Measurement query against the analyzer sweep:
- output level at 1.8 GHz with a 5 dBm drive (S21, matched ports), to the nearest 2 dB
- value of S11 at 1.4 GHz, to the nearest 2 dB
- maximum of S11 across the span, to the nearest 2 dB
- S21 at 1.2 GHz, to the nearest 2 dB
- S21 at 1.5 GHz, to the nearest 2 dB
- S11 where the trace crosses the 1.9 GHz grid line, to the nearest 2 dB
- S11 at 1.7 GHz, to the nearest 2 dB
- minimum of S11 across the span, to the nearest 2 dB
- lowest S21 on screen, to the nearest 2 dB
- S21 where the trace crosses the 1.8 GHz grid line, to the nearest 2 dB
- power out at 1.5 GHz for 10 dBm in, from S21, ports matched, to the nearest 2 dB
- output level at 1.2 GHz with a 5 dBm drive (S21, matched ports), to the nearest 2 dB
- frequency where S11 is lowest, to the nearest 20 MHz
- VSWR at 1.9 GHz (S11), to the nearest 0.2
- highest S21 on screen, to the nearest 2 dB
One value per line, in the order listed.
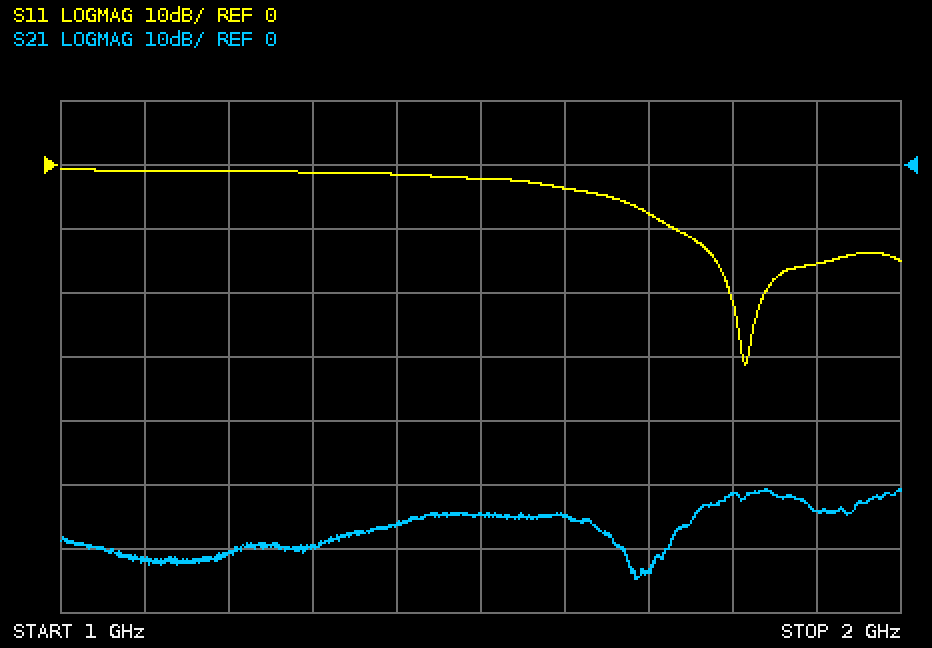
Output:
-46 dBm
-2 dB
0 dB
-60 dB
-54 dB
-16 dB
-8 dB
-32 dB
-64 dB
-52 dB
-44 dBm
-56 dBm
1.82 GHz
1.4
-50 dB
